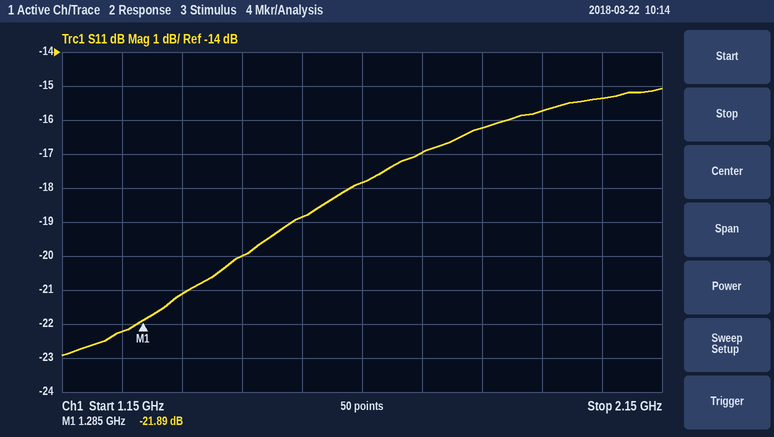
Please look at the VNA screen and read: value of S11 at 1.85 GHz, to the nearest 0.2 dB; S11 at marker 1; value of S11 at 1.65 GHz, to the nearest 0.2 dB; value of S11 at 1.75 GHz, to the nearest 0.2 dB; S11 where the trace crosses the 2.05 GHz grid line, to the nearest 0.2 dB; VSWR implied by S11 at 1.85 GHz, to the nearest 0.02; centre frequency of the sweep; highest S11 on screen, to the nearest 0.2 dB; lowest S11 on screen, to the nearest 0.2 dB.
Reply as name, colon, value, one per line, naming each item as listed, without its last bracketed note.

value of S11 at 1.85 GHz, to the nearest 0.2 dB: -16.2 dB
S11 at marker 1: -21.89 dB
value of S11 at 1.65 GHz, to the nearest 0.2 dB: -17.8 dB
value of S11 at 1.75 GHz, to the nearest 0.2 dB: -17.0 dB
S11 where the trace crosses the 2.05 GHz grid line, to the nearest 0.2 dB: -15.4 dB
VSWR implied by S11 at 1.85 GHz, to the nearest 0.02: 1.36
centre frequency of the sweep: 1.65 GHz
highest S11 on screen, to the nearest 0.2 dB: -15.0 dB
lowest S11 on screen, to the nearest 0.2 dB: -23.0 dB
